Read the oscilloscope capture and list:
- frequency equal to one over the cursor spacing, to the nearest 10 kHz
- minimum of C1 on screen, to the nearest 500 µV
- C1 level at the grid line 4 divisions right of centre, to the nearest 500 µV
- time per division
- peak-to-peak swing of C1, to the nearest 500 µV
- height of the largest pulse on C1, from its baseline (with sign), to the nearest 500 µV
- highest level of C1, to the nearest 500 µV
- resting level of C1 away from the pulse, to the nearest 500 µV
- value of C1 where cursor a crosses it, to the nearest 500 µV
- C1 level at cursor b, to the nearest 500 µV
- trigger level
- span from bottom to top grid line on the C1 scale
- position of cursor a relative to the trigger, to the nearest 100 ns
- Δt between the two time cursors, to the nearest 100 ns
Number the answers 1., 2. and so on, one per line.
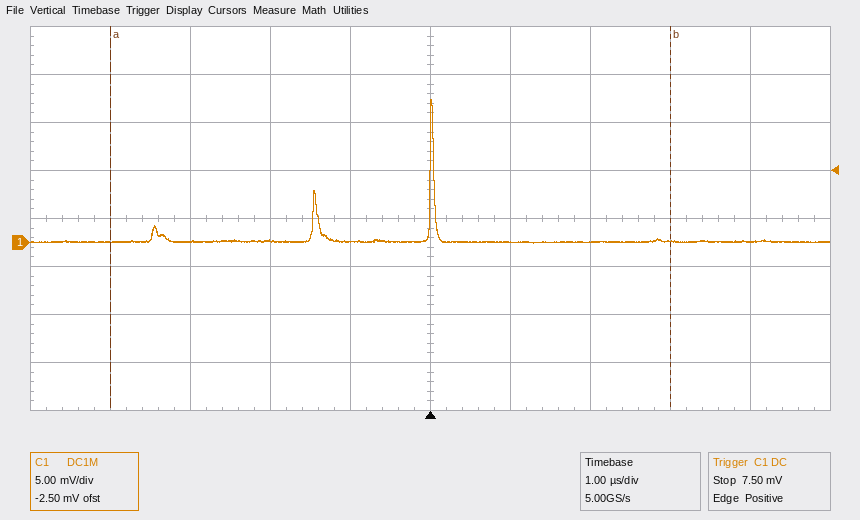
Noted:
1. 140 kHz
2. 0.0 mV
3. 0.0 mV
4. 1 µs
5. 15.0 mV
6. +15.0 mV
7. 15.0 mV
8. 0.0 mV
9. 0.0 mV
10. 0.0 mV
11. 7.50 mV
12. 40 mV
13. -4.0 µs
14. 7.0 µs
